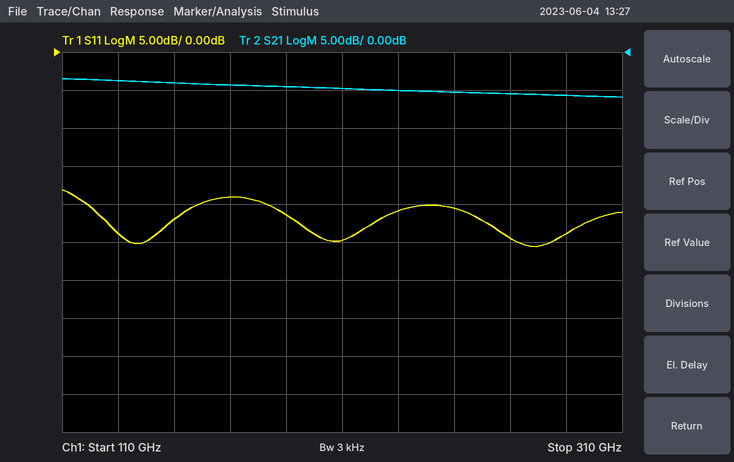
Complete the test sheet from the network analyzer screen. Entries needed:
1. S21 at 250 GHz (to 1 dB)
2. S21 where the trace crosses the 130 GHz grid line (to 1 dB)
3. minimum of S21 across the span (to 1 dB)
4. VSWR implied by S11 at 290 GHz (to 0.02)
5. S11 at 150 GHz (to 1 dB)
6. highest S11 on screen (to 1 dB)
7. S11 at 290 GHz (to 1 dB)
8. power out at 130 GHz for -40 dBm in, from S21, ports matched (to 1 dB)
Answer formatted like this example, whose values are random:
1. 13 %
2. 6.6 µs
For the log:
1. -5 dB
2. -4 dB
3. -6 dB
4. 1.14
5. -22 dB
6. -18 dB
7. -24 dB
8. -44 dBm
